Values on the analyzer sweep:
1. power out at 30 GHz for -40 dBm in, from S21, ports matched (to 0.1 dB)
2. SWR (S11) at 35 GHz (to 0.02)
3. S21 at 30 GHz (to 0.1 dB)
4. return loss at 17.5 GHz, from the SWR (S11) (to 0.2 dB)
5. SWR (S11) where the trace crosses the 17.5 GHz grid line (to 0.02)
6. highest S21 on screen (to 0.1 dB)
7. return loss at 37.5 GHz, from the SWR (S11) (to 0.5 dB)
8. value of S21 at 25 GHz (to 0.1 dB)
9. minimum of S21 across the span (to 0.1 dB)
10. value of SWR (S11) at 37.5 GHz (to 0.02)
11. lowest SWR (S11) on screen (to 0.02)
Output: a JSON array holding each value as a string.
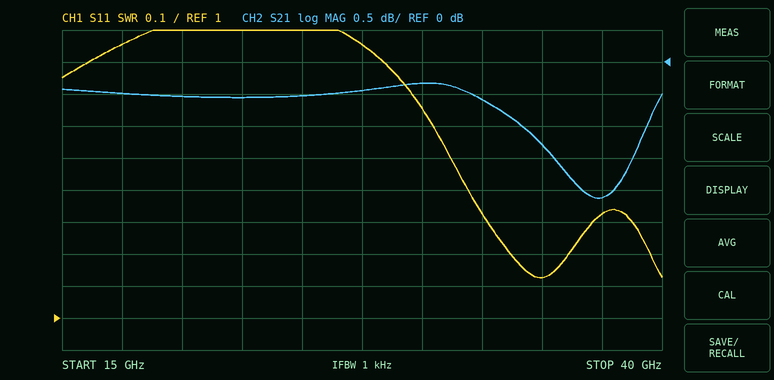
["-40.3 dBm", "1.12", "-0.3 dB", "10.4 dB", "1.86", "-0.3 dB", "17.0 dB", "-0.5 dB", "-2.1 dB", "1.32", "1.12"]
